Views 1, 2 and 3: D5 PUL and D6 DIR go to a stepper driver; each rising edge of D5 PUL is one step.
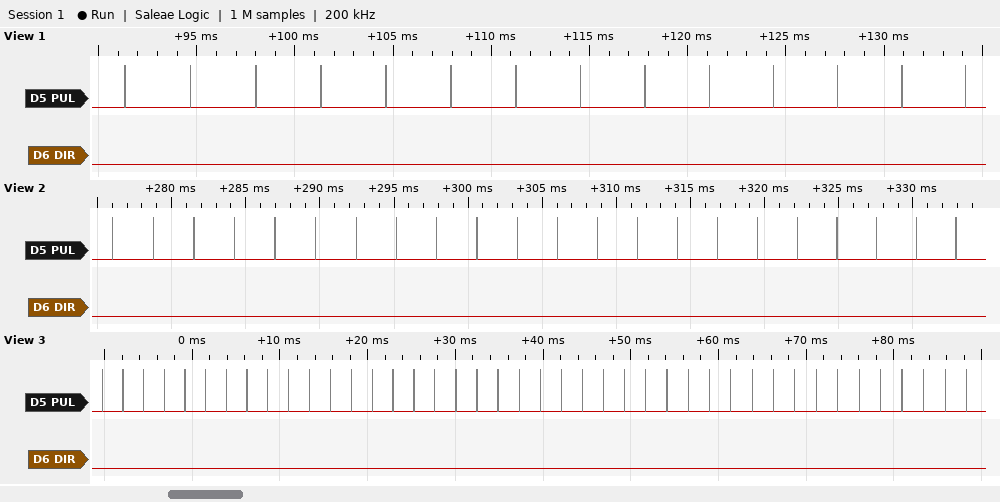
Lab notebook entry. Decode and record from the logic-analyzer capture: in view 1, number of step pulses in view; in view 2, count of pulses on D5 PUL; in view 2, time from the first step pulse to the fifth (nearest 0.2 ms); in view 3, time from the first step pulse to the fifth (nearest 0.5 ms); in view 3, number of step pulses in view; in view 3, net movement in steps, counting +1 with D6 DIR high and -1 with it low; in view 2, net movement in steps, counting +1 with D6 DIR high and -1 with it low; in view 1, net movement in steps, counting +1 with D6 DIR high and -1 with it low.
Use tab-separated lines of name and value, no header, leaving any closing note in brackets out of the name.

in view 1, number of step pulses in view	14
in view 2, count of pulses on D5 PUL	22
in view 2, time from the first step pulse to the fifth	11.0 ms
in view 3, time from the first step pulse to the fifth	9.5 ms
in view 3, number of step pulses in view	42
in view 3, net movement in steps, counting +1 with D6 DIR high and -1 with it low	-42
in view 2, net movement in steps, counting +1 with D6 DIR high and -1 with it low	-22
in view 1, net movement in steps, counting +1 with D6 DIR high and -1 with it low	-14
